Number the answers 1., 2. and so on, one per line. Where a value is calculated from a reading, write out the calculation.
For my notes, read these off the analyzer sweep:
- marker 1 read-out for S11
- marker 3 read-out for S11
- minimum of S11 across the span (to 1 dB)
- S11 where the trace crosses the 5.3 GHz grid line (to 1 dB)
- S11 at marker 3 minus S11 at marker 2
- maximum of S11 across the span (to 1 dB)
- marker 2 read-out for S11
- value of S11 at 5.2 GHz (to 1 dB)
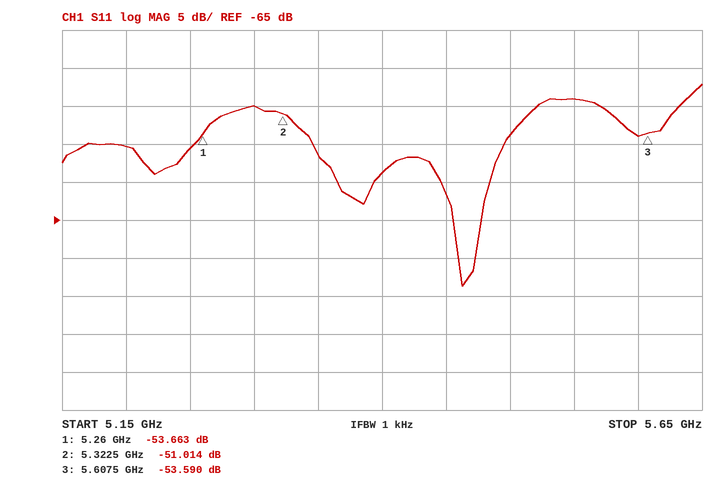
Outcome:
1. -53.663 dB
2. -53.590 dB
3. -74 dB
4. -50 dB
5. -53.59 − (-51.014) = -2.576 dB
6. -47 dB
7. -51.014 dB
8. -55 dB
